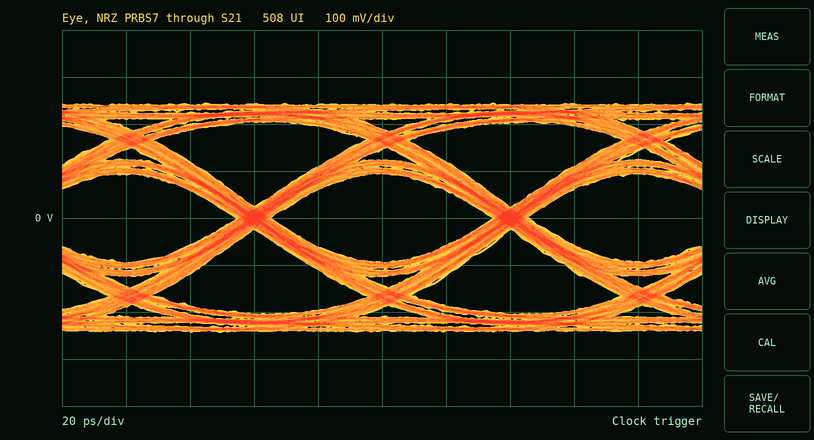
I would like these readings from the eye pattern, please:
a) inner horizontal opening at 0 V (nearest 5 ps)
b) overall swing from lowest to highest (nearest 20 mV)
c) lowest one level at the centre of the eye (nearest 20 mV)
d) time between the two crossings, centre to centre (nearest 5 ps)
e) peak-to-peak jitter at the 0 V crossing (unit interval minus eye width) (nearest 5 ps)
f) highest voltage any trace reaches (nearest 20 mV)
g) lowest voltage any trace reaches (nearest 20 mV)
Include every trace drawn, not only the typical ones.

70 ps
480 mV
100 mV
80 ps
10 ps
240 mV
-240 mV
